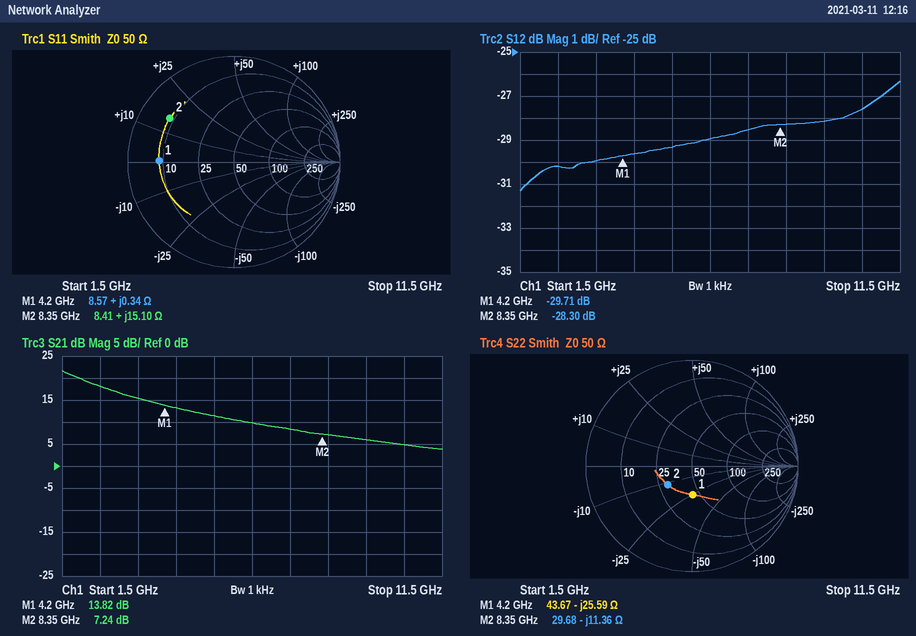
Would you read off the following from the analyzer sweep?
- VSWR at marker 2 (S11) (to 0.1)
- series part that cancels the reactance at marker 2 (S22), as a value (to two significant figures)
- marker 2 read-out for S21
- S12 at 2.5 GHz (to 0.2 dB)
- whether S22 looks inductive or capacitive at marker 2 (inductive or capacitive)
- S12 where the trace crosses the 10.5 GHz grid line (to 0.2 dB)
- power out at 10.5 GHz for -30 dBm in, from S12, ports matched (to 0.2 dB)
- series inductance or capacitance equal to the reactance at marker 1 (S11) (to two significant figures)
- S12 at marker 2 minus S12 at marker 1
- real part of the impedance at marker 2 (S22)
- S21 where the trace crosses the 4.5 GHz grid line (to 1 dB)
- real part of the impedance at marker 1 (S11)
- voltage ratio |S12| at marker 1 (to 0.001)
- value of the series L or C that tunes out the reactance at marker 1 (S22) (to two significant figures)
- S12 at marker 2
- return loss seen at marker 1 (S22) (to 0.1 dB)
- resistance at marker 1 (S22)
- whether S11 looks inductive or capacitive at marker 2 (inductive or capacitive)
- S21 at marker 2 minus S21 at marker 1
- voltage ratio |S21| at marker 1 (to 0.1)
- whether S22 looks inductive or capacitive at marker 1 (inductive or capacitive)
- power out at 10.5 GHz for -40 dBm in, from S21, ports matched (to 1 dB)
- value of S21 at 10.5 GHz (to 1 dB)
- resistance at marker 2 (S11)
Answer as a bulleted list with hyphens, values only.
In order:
- 6.5
- 220 pH
- 7.24 dB
- -30.2 dB
- capacitive
- -27.6 dB
- -57.6 dBm
- 13 pH
- 1.41 dB
- 29.68 Ω
- 13 dB
- 8.57 Ω
- 0.033
- 970 pH
- -28.30 dB
- 11.3 dB
- 43.67 Ω
- inductive
- -6.58 dB
- 4.9
- capacitive
- -35 dBm
- 5 dB
- 8.41 Ω
